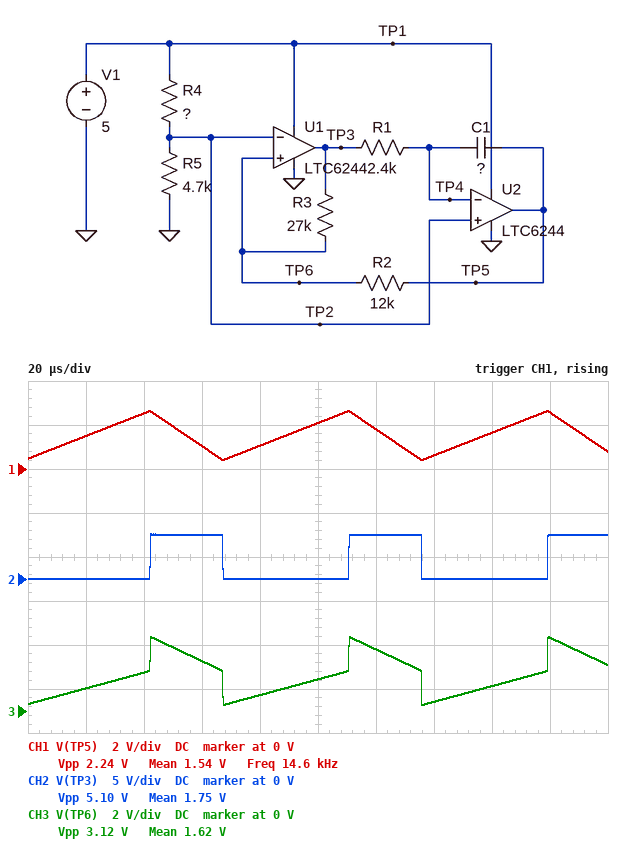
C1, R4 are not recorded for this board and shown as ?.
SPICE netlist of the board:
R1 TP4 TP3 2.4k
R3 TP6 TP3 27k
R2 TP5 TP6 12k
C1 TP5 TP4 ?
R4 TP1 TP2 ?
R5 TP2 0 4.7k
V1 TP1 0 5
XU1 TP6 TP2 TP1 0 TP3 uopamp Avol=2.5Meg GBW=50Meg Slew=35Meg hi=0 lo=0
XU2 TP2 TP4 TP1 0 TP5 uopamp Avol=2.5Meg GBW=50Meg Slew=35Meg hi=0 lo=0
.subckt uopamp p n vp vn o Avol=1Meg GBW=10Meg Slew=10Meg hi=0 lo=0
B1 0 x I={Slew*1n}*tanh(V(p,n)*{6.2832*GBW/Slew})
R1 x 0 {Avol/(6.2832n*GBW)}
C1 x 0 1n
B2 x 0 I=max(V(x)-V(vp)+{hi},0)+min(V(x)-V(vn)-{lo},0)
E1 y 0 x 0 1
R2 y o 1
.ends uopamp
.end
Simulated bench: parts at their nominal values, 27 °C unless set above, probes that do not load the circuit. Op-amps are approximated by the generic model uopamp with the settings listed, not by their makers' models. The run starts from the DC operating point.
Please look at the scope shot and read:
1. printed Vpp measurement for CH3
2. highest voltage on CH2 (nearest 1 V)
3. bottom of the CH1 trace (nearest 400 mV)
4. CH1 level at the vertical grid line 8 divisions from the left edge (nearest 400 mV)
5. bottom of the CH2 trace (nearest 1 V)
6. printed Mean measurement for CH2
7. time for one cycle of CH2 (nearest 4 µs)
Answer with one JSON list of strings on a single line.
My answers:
["3.12 V", "5 V", "400 mV", "1.6 V", "0 V", "1.75 V", "68 µs"]
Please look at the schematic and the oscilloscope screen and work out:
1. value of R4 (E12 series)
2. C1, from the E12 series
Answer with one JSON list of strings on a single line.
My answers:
["8.2 kΩ", "15 nF"]
